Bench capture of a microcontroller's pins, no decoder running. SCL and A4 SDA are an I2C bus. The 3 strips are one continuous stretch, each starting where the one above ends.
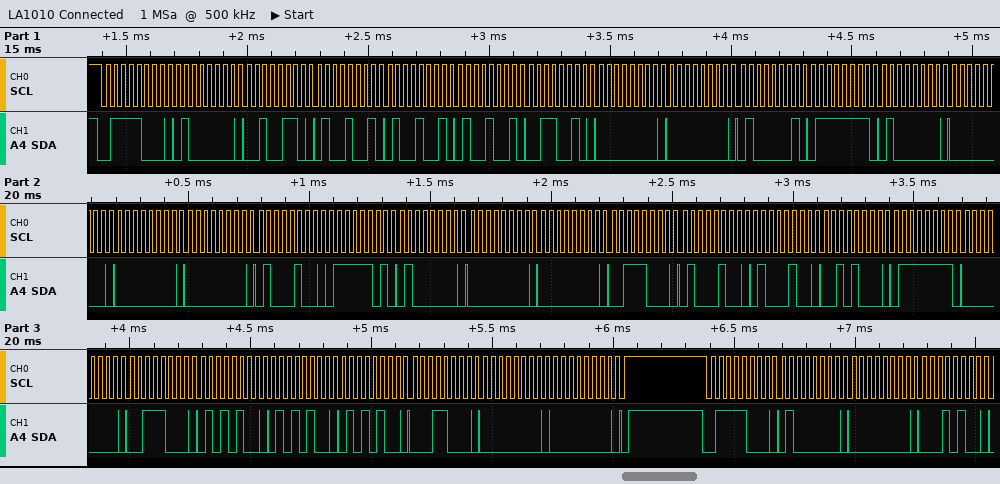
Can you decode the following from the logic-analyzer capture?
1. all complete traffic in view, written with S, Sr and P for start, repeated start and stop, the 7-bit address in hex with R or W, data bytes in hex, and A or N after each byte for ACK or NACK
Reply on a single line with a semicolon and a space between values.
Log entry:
S 3CW A 40 A 26 A 49 A 49 A 49 A 32 A 00 A 00 A 41 A 7F A 40 A 00 A 00 A 00 A 44 A 7D A 40 A 00 A 00 A 38 A 44 A 44 A 28 A 7F A 00 A 38 A 54 A 54 A 54 A 18 A 00 A 00 A P S 3CW A 40 A 00 A 14 A
